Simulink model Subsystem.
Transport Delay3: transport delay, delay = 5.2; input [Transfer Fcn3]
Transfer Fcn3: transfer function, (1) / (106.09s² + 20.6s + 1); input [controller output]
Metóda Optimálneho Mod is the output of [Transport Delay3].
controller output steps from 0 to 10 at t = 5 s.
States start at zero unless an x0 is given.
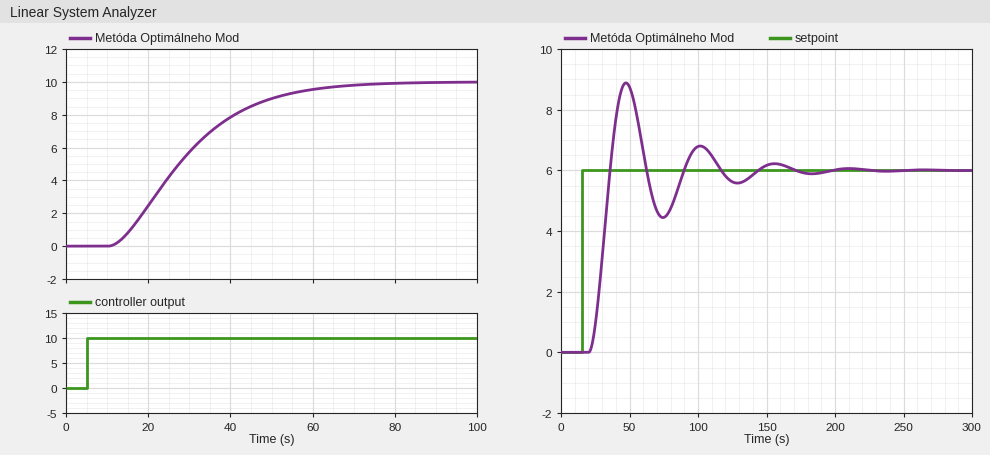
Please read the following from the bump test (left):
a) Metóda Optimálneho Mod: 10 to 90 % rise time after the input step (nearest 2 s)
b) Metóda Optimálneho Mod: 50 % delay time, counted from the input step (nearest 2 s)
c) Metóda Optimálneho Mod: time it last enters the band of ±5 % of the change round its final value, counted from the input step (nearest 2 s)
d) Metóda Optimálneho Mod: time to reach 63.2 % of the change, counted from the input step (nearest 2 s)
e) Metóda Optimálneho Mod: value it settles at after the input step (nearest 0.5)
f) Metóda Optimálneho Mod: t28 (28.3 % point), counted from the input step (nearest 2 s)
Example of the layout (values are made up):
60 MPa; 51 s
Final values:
34 s; 22 s; 54 s; 28 s; 10.0; 16 s
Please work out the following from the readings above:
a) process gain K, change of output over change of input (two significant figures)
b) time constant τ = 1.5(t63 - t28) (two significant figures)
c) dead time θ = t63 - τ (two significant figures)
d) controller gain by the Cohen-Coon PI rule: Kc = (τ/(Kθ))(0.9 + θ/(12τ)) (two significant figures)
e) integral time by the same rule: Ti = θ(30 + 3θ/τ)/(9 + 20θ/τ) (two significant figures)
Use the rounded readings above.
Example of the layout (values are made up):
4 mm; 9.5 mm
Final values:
1.0; 18 s; 10 s; 1.7; 16 s
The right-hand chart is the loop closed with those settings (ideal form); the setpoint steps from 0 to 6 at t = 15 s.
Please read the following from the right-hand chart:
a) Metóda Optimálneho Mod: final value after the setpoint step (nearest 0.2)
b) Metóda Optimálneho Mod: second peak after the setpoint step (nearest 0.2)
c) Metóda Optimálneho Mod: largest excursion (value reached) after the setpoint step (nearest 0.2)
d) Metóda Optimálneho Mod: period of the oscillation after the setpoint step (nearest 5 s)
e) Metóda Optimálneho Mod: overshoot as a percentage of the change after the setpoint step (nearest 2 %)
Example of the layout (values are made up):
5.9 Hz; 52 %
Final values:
6.0; 6.8; 8.8; 55 s; 48 %
